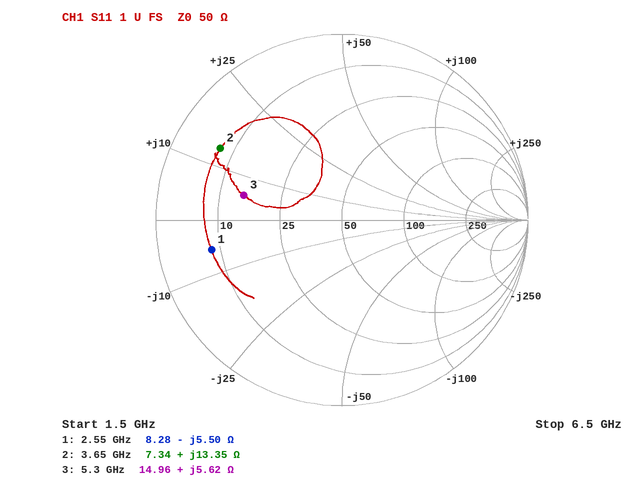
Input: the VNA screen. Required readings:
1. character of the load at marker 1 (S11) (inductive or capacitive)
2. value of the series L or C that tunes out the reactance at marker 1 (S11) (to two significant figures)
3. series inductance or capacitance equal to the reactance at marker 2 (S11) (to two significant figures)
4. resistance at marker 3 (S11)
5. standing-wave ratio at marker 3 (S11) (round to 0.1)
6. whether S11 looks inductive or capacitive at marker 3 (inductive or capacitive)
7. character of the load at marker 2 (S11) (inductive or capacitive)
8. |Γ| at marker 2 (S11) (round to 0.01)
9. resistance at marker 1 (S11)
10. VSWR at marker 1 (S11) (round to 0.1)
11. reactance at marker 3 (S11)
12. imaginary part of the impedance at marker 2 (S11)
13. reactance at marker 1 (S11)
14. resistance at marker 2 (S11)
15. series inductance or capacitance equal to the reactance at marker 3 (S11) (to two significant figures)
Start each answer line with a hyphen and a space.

- capacitive
- 340 pH
- 580 pH
- 14.96 Ω
- 3.4
- inductive
- inductive
- 0.76
- 8.28 Ω
- 6.1
- +5.62 Ω
- +13.35 Ω
- -5.50 Ω
- 7.34 Ω
- 170 pH
